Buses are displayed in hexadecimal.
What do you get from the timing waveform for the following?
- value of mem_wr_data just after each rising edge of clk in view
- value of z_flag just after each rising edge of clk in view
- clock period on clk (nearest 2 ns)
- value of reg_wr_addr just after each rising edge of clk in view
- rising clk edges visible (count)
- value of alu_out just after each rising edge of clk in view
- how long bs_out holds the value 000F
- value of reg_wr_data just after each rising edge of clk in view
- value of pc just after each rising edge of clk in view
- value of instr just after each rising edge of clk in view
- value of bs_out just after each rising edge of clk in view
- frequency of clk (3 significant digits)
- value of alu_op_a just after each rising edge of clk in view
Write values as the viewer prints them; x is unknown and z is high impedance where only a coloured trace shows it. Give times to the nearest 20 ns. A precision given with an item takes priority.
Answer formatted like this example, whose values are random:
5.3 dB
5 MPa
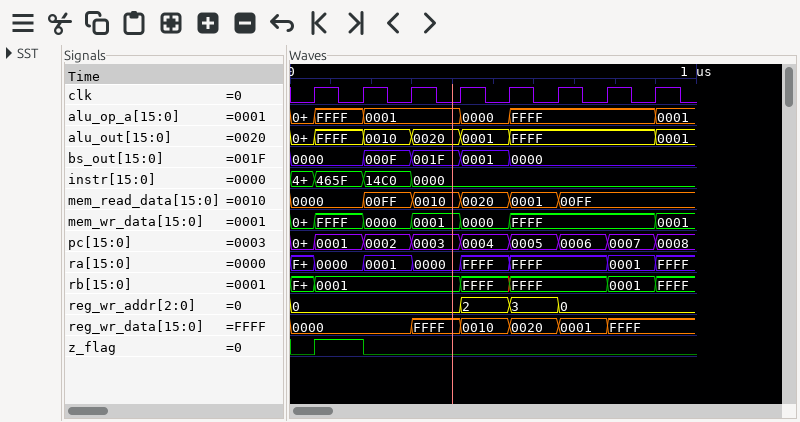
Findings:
FFFF, 0000, 0001, 0000, FFFF, FFFF, FFFF, 0001
1 0 0 0 0 0 0 0
120 ns
0, 0, 0, 2, 3, 0, 0, 0
8
FFFF, 0010, 0020, 0001, FFFF, FFFF, FFFF, 0001
120 ns
0000, 0000, FFFF, 0010, 0020, 0001, FFFF, FFFF
0001, 0002, 0003, 0004, 0005, 0006, 0007, 0008
465F, 14C0, 0000, 0000, 0000, 0000, 0000, 0000
0000, 000F, 001F, 0001, 0000, 0000, 0000, 0000
8.33 MHz
FFFF, 0001, 0001, 0000, FFFF, FFFF, FFFF, 0001
